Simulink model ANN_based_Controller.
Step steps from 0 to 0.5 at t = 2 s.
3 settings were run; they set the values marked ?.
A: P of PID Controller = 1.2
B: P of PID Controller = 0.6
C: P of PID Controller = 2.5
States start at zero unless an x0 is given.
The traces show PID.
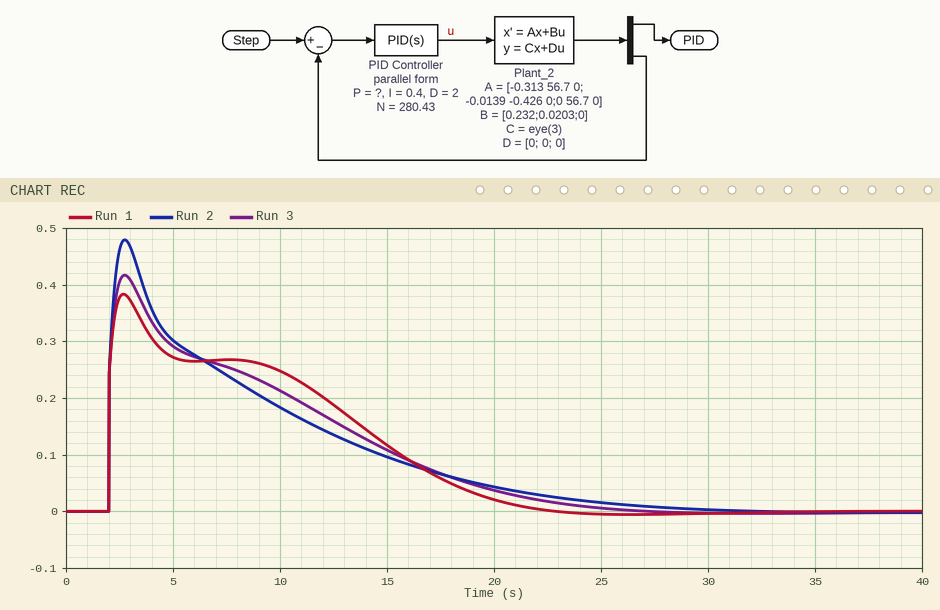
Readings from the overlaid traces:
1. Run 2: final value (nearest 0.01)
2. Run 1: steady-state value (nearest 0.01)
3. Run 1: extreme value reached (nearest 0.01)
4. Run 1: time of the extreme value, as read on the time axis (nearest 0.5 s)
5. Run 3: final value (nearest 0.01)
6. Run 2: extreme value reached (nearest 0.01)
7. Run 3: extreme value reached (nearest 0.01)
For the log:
0.00
0.00
0.38
2.5 s
0.00
0.48
0.42
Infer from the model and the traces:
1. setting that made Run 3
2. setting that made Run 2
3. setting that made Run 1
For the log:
A
C
B
